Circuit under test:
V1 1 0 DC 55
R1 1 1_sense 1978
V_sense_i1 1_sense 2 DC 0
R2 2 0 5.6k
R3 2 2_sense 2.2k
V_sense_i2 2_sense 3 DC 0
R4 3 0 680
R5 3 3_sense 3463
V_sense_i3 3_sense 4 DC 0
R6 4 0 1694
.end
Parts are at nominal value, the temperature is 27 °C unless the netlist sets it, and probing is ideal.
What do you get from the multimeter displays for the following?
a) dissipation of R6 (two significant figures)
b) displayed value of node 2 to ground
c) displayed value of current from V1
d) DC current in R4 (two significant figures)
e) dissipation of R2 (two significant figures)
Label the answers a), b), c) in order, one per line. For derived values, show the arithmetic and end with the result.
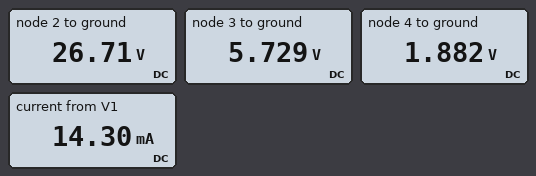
a) (1.882 V)^2 / 1.694 kΩ = 2.1 mW
b) 26.71 V
c) 14.30 mA
d) (5.729 V) / 680 Ω = 8.4 mA
e) (26.71 V)^2 / 5.6 kΩ = 130 mW
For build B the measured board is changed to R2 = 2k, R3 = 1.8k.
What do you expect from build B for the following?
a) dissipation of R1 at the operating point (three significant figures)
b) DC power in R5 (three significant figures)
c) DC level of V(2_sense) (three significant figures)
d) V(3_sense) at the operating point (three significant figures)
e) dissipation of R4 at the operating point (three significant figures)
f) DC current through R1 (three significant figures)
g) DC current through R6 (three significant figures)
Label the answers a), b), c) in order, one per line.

a) 635 mW
b) 3.12 mW
c) 4.89 V
d) 1.61 V
e) 35.2 mW
f) 17.9 mA
g) 949 µA
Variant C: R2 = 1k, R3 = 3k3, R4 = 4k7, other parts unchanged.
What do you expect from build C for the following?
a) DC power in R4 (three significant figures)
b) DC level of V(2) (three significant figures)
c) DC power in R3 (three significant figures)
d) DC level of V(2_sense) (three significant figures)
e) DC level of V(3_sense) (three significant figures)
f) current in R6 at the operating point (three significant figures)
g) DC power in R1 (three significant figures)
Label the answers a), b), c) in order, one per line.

a) 10.6 mW
b) 16.6 V
c) 27.3 mW
d) 7.07 V
e) 2.32 V
f) 1.37 mA
g) 747 mW
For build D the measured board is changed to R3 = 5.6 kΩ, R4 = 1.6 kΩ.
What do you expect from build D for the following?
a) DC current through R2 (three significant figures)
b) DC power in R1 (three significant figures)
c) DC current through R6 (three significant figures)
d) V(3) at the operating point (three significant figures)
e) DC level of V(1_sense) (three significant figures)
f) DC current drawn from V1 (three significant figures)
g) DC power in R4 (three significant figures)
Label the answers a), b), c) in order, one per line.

a) 5.98 mA
b) 234 mW
c) 1.16 mA
d) 5.99 V
e) 33.5 V
f) 10.9 mA
g) 22.4 mW
